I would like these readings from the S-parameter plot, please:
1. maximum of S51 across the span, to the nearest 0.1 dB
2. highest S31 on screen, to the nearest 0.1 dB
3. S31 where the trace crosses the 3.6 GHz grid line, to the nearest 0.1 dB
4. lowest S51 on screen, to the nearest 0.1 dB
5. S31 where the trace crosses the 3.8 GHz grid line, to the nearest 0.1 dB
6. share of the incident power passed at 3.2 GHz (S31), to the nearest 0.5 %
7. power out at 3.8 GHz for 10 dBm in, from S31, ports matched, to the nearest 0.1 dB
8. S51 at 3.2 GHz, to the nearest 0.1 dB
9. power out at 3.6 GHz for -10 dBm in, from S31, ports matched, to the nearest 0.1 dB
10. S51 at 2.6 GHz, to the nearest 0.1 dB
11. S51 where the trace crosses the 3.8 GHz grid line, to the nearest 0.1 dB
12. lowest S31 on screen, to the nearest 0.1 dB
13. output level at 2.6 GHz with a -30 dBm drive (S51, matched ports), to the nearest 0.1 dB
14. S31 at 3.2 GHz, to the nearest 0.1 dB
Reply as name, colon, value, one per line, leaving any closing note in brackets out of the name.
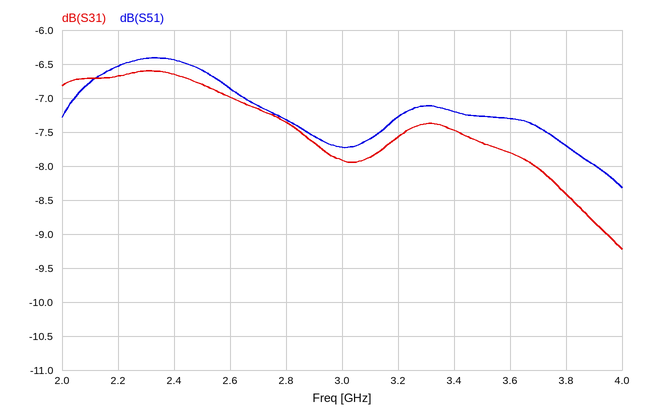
maximum of S51 across the span, to the nearest 0.1 dB: -6.4 dB
highest S31 on screen, to the nearest 0.1 dB: -6.6 dB
S31 where the trace crosses the 3.6 GHz grid line, to the nearest 0.1 dB: -7.8 dB
lowest S51 on screen, to the nearest 0.1 dB: -8.3 dB
S31 where the trace crosses the 3.8 GHz grid line, to the nearest 0.1 dB: -8.4 dB
share of the incident power passed at 3.2 GHz (S31), to the nearest 0.5 %: 17.5 %
power out at 3.8 GHz for 10 dBm in, from S31, ports matched, to the nearest 0.1 dB: 1.6 dBm
S51 at 3.2 GHz, to the nearest 0.1 dB: -7.3 dB
power out at 3.6 GHz for -10 dBm in, from S31, ports matched, to the nearest 0.1 dB: -17.8 dBm
S51 at 2.6 GHz, to the nearest 0.1 dB: -6.9 dB
S51 where the trace crosses the 3.8 GHz grid line, to the nearest 0.1 dB: -7.7 dB
lowest S31 on screen, to the nearest 0.1 dB: -9.2 dB
output level at 2.6 GHz with a -30 dBm drive (S51, matched ports), to the nearest 0.1 dB: -36.9 dBm
S31 at 3.2 GHz, to the nearest 0.1 dB: -7.6 dB
